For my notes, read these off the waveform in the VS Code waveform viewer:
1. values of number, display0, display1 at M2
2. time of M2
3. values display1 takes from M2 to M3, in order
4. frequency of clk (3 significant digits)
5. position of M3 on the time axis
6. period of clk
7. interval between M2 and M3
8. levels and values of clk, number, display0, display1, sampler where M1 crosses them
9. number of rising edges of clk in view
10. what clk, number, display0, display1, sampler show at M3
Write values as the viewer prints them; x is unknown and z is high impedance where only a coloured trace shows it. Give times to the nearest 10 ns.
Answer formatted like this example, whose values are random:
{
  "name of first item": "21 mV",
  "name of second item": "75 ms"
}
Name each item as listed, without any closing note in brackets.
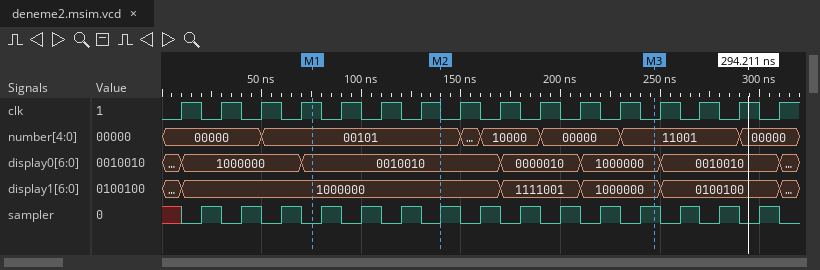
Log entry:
{
  "values of number, display0, display1 at M2": "number=00101, display0=0010010, display1=1000000",
  "time of M2": "140 ns",
  "values display1 takes from M2 to M3, in order": "1000000, 1111001, 1000000",
  "frequency of clk": "50.0 MHz",
  "position of M3 on the time axis": "250 ns",
  "period of clk": "20 ns",
  "interval between M2 and M3": "110 ns",
  "levels and values of clk, number, display0, display1, sampler where M1 crosses them": "clk=1, number=00101, display0=0010010, display1=1000000, sampler=0",
  "number of rising edges of clk in view": "16",
  "what clk, number, display0, display1, sampler show at M3": "clk=0, number=11001, display0=1000000, display1=1000000, sampler=1"
}
